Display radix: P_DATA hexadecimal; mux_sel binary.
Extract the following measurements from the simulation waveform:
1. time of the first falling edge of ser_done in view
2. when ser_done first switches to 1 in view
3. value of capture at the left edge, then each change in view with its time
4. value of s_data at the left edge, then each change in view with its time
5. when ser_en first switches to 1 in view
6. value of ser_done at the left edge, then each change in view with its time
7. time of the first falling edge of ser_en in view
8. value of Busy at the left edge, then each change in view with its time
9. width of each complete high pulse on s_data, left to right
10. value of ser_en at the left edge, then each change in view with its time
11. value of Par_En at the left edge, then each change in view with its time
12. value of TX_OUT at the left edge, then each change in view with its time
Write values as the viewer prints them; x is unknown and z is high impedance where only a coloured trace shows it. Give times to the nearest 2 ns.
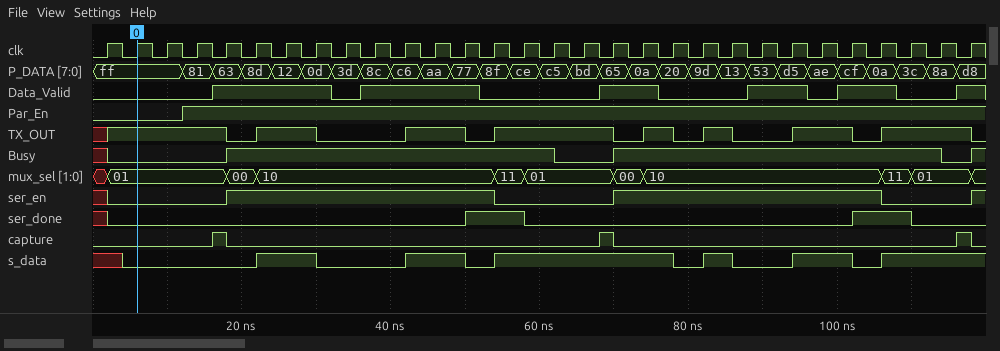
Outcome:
58 ns
50 ns
0, 1 at 16 ns, 0 at 18 ns, 1 at 68 ns, 0 at 70 ns, 1 at 116 ns, 0 at 118 ns
x, 0 at 4 ns, 1 at 22 ns, 0 at 30 ns, 1 at 42 ns, 0 at 50 ns, 1 at 54 ns, 0 at 78 ns, 1 at 82 ns, 0 at 86 ns, 1 at 94 ns, 0 at 102 ns, 1 at 106 ns
18 ns
x, 0 at 2 ns, 1 at 50 ns, 0 at 58 ns, 1 at 102 ns, 0 at 110 ns
54 ns
x, 0 at 2 ns, 1 at 18 ns, 0 at 62 ns, 1 at 70 ns, 0 at 114 ns, 1 at 118 ns
8 ns, 8 ns, 24 ns, 4 ns, 8 ns
x, 0 at 2 ns, 1 at 18 ns, 0 at 54 ns, 1 at 70 ns, 0 at 106 ns, 1 at 118 ns
0, 1 at 12 ns
x, 1 at 2 ns, 0 at 18 ns, 1 at 22 ns, 0 at 30 ns, 1 at 42 ns, 0 at 50 ns, 1 at 54 ns, 0 at 70 ns, 1 at 74 ns, 0 at 78 ns, 1 at 82 ns, 0 at 86 ns, 1 at 94 ns, 0 at 102 ns, 1 at 106 ns, 0 at 118 ns
